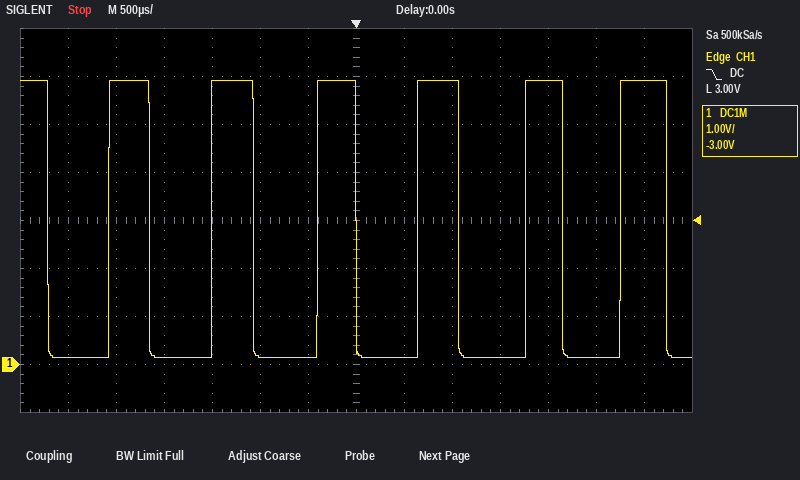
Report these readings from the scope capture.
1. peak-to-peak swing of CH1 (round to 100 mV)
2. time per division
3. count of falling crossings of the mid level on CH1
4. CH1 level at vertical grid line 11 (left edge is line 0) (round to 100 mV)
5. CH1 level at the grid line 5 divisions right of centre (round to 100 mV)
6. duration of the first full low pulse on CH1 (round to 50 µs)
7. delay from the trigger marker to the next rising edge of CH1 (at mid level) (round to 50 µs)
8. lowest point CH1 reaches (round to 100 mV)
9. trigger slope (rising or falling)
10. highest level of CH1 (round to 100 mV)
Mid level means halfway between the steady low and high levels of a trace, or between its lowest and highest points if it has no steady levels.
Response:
5.8 V
500 µs
7
5.9 V
100 mV
650 µs
650 µs
100 mV
falling
5.9 V
